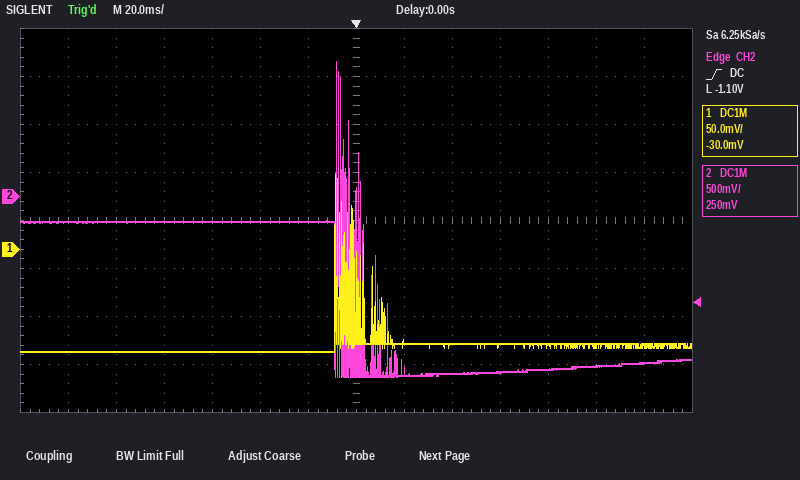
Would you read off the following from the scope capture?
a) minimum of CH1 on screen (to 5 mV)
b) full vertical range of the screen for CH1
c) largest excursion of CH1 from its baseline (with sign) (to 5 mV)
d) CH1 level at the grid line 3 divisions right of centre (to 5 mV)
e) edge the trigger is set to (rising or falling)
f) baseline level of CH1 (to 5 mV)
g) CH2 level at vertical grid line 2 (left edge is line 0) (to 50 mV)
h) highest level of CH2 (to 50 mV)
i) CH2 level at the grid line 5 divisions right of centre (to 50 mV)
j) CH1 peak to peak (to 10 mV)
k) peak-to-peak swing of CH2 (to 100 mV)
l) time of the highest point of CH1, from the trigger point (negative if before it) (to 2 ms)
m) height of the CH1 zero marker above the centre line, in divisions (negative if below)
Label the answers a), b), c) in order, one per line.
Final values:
a) -105 mV
b) 400 mV
c) +175 mV
d) -100 mV
e) rising
f) -100 mV
g) -250 mV
h) 1.40 V
i) -1.75 V
j) 180 mV
k) 3.30 V
l) -8 ms
m) -0.6 div
